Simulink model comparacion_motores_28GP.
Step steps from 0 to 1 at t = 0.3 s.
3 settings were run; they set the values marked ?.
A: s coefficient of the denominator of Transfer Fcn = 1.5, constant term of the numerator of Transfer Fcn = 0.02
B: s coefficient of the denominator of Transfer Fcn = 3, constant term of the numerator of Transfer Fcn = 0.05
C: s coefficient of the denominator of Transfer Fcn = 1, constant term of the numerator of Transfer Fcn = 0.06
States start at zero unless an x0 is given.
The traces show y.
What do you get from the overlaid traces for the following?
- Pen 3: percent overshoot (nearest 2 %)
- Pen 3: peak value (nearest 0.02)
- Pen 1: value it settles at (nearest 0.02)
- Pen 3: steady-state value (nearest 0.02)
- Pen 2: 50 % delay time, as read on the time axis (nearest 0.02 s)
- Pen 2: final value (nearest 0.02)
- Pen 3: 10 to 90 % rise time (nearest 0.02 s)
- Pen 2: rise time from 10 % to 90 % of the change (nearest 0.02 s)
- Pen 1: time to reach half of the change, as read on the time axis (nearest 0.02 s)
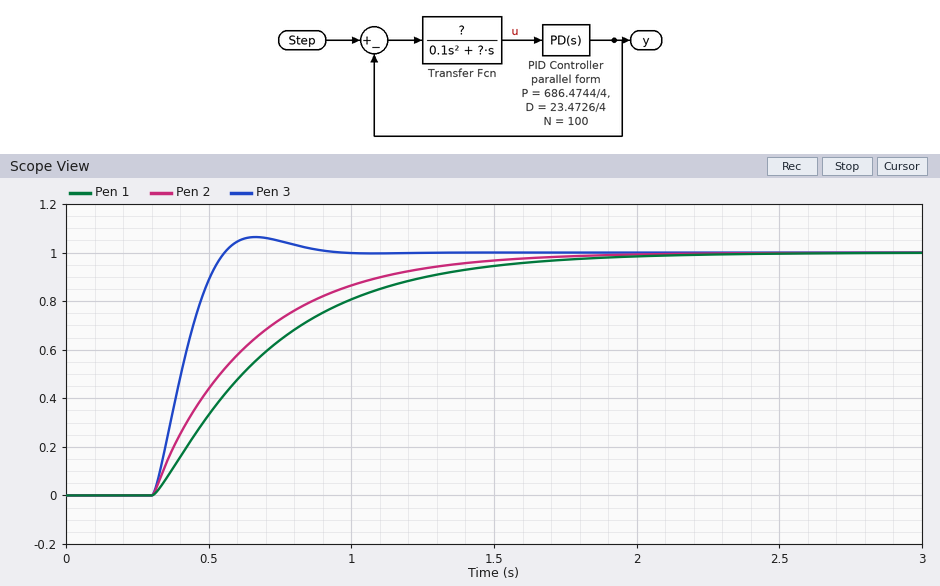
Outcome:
6 %
1.06
1.00
1.00
0.54 s
1.00
0.18 s
0.76 s
0.62 s
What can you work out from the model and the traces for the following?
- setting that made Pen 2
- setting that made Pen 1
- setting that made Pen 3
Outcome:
B
A
C
